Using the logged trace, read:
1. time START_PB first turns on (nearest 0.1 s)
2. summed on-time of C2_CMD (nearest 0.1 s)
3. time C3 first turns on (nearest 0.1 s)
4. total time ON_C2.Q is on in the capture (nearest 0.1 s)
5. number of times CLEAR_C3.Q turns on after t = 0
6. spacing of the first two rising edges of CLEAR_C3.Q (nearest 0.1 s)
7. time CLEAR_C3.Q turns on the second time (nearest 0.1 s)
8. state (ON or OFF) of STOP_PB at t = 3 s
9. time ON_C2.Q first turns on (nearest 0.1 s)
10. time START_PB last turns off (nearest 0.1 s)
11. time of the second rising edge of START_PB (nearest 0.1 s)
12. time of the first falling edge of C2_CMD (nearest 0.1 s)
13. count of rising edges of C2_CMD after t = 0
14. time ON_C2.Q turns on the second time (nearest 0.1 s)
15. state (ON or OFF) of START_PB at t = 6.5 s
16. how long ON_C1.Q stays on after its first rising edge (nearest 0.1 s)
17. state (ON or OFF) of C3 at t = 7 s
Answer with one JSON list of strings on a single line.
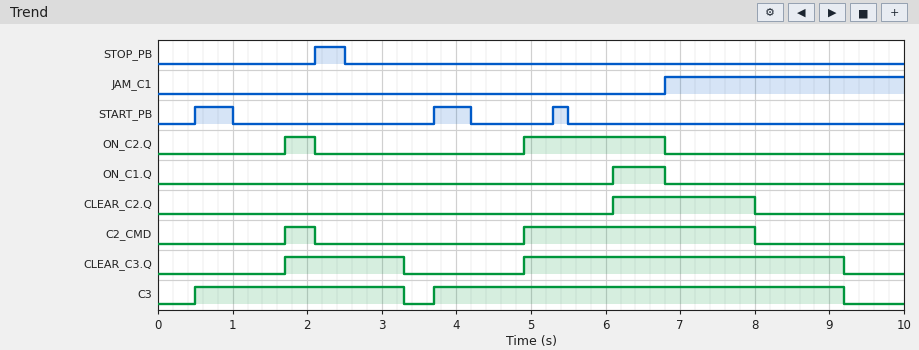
["0.5 s", "3.5 s", "0.5 s", "2.3 s", "2", "3.2 s", "4.9 s", "OFF", "1.7 s", "5.5 s", "3.7 s", "2.1 s", "2", "4.9 s", "OFF", "0.7 s", "ON"]
